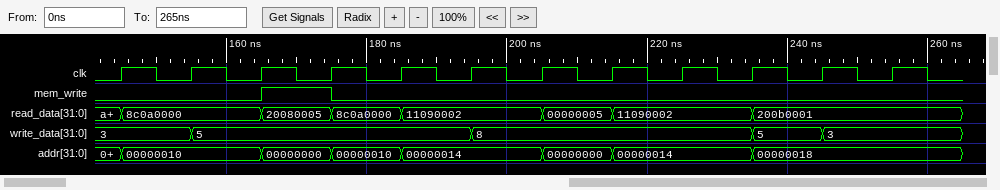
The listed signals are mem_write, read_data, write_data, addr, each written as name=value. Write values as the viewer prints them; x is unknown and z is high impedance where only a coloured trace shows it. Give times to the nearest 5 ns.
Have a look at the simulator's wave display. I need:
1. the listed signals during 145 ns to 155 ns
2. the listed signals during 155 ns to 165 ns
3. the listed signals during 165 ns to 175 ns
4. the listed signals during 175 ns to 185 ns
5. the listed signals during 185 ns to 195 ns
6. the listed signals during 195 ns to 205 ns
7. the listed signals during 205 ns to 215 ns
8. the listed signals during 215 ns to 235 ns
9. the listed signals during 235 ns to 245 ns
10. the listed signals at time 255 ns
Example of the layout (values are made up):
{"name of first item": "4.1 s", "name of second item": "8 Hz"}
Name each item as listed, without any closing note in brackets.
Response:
{"the listed signals during 145 ns to 155 ns": "mem_write=0, read_data=8c0a0000, write_data=3, addr=00000010", "the listed signals during 155 ns to 165 ns": "mem_write=0, read_data=8c0a0000, write_data=5, addr=00000010", "the listed signals during 165 ns to 175 ns": "mem_write=1, read_data=20080005, write_data=5, addr=00000000", "the listed signals during 175 ns to 185 ns": "mem_write=0, read_data=8c0a0000, write_data=5, addr=00000010", "the listed signals during 185 ns to 195 ns": "mem_write=0, read_data=11090002, write_data=5, addr=00000014", "the listed signals during 195 ns to 205 ns": "mem_write=0, read_data=11090002, write_data=8, addr=00000014", "the listed signals during 205 ns to 215 ns": "mem_write=0, read_data=00000005, write_data=8, addr=00000000", "the listed signals during 215 ns to 235 ns": "mem_write=0, read_data=11090002, write_data=8, addr=00000014", "the listed signals during 235 ns to 245 ns": "mem_write=0, read_data=200b0001, write_data=5, addr=00000018", "the listed signals at time 255 ns": "mem_write=0, read_data=200b0001, write_data=3, addr=00000018"}
